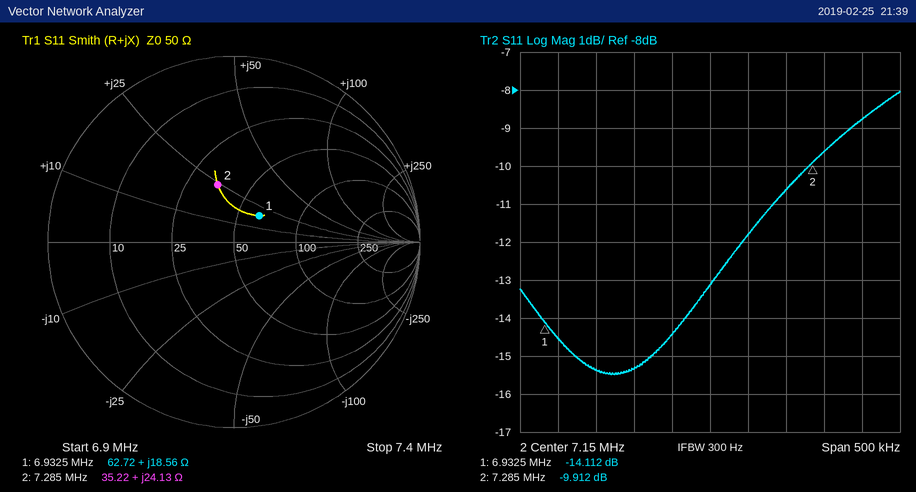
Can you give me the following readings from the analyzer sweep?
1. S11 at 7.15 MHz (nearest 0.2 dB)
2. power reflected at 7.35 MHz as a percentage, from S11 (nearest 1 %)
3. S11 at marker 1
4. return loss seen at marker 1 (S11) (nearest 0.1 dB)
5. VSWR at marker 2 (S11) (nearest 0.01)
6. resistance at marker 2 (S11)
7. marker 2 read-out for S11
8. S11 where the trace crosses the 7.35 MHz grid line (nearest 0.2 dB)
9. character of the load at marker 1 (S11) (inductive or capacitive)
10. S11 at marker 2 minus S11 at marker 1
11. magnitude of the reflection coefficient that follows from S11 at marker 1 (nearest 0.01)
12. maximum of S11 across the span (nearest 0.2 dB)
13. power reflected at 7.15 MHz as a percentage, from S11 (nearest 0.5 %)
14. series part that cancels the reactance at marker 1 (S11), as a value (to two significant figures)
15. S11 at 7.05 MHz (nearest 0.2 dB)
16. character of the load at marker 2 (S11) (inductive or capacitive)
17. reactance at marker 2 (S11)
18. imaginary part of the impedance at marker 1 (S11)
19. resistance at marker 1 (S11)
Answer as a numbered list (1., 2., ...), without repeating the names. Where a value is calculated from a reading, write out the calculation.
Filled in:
1. -13.2 dB
2. 10^(-8.8/10) ≈ 13 %
3. -14.112 dB
4. 14.1 dB
5. 1.94
6. 35.22 Ω
7. -9.912 dB
8. -8.8 dB
9. inductive
10. -9.912 − (-14.112) = 4.200 dB
11. 10^(-14.112/20) ≈ 0.20
12. -8.0 dB
13. 10^(-13.2/10) ≈ 4.79 %, so 5.0 % to the nearest 0.5 %
14. C = 1/(2π × 6.9325 MHz × 18.56 Ω) ≈ 1.2 nF
15. -15.4 dB
16. inductive
17. +24.13 Ω
18. +18.56 Ω
19. 62.72 Ω
